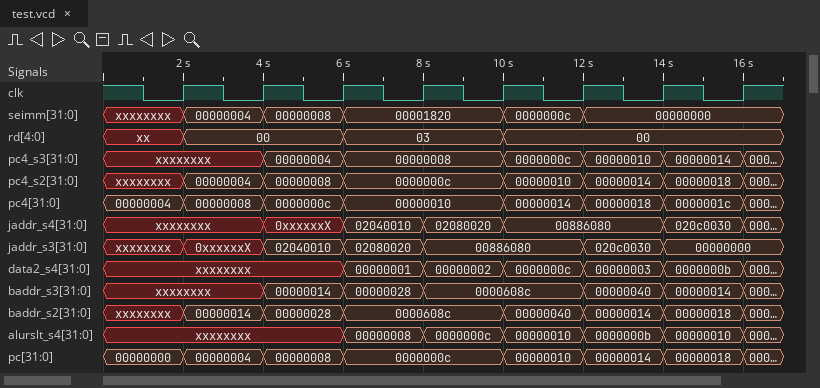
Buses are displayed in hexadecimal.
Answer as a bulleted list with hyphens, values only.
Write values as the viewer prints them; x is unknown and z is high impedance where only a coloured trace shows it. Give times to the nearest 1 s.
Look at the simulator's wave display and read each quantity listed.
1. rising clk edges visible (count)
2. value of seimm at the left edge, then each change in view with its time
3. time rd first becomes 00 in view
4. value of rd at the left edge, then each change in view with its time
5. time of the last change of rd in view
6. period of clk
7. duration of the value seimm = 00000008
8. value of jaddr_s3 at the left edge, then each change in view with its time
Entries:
- 8
- xxxxxxxx, 00000004 at 2 s, 00000008 at 4 s, 00001820 at 6 s, 0000000c at 10 s, 00000000 at 12 s
- 2 s
- xx, 00 at 2 s, 03 at 6 s, 00 at 10 s
- 10 s
- 2 s
- 2 s
- xxxxxxxx, 0xxxxxxX at 2 s, 02040010 at 4 s, 02080020 at 6 s, 00886080 at 8 s, 020c0030 at 12 s, 00000000 at 14 s
